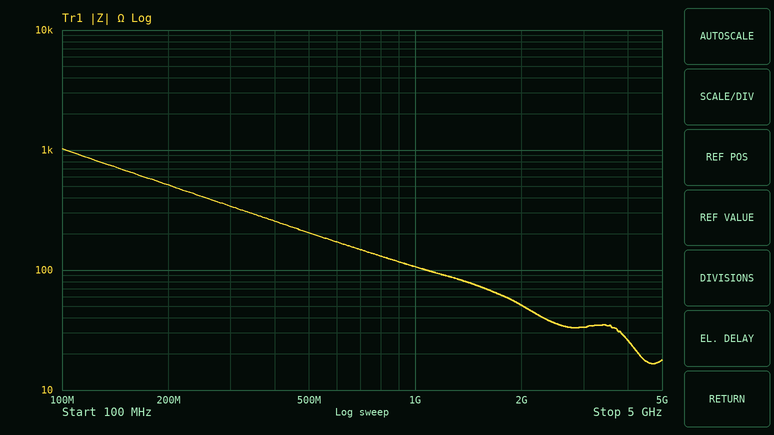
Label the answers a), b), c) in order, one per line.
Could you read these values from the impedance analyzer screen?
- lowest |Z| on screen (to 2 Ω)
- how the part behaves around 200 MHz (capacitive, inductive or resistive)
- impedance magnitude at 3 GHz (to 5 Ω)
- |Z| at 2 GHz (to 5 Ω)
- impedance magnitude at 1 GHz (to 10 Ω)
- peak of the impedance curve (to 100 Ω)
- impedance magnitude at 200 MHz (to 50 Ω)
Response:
a) 16 Ω
b) capacitive
c) 35 Ω
d) 50 Ω
e) 110 Ω
f) 1.0 kΩ
g) 500 Ω
